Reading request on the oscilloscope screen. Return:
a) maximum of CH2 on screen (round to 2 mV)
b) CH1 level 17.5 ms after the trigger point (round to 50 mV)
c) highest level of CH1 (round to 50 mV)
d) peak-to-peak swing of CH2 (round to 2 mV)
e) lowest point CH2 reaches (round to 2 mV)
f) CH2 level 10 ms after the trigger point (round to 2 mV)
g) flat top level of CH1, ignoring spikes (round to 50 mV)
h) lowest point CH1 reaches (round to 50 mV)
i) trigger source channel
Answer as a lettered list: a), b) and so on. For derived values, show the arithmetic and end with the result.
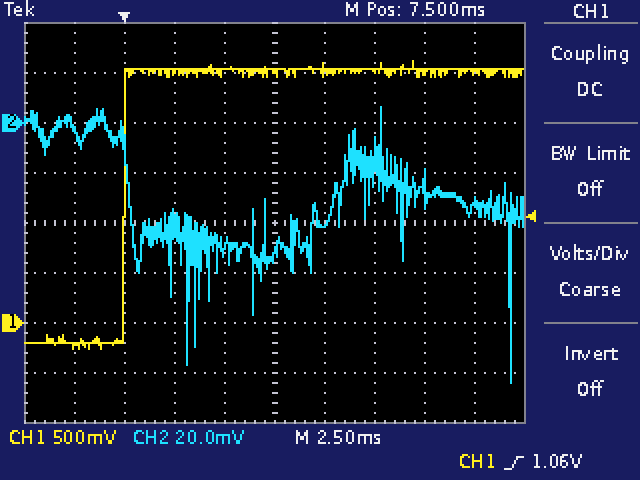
a) 6 mV
b) 2.50 V
c) 2.60 V
d) 6 mV − (-104 mV) = 110 mV
e) -104 mV
f) -40 mV
g) 2.55 V
h) -250 mV
i) CH1
